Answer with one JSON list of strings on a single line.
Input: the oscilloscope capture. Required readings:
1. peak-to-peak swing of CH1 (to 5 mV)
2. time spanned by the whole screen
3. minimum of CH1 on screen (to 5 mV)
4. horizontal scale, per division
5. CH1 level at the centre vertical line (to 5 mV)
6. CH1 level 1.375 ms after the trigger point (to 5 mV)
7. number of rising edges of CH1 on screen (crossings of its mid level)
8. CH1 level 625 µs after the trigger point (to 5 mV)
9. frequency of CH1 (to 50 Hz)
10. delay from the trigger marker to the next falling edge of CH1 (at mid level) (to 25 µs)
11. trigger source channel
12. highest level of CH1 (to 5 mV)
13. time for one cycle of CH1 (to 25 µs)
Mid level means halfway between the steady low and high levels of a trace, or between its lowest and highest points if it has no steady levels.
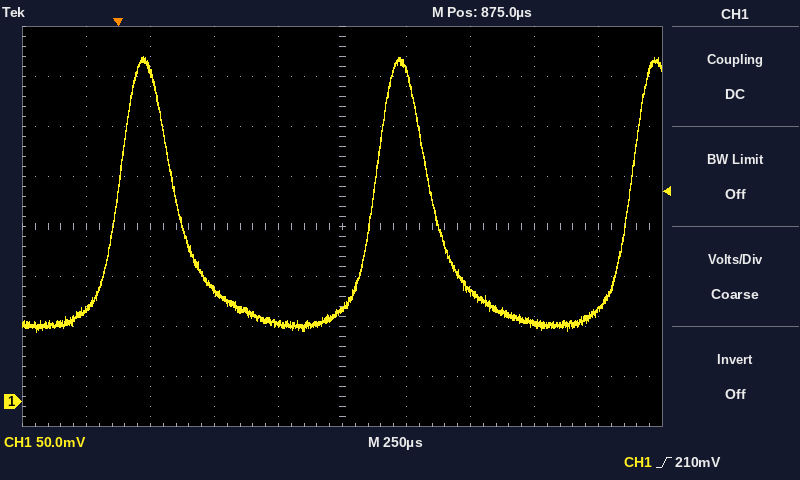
["275 mV", "2.5 ms", "70 mV", "250 µs", "95 mV", "110 mV", "3", "80 mV", "1.00 kHz", "225 µs", "CH1", "345 mV", "1.000 ms"]
